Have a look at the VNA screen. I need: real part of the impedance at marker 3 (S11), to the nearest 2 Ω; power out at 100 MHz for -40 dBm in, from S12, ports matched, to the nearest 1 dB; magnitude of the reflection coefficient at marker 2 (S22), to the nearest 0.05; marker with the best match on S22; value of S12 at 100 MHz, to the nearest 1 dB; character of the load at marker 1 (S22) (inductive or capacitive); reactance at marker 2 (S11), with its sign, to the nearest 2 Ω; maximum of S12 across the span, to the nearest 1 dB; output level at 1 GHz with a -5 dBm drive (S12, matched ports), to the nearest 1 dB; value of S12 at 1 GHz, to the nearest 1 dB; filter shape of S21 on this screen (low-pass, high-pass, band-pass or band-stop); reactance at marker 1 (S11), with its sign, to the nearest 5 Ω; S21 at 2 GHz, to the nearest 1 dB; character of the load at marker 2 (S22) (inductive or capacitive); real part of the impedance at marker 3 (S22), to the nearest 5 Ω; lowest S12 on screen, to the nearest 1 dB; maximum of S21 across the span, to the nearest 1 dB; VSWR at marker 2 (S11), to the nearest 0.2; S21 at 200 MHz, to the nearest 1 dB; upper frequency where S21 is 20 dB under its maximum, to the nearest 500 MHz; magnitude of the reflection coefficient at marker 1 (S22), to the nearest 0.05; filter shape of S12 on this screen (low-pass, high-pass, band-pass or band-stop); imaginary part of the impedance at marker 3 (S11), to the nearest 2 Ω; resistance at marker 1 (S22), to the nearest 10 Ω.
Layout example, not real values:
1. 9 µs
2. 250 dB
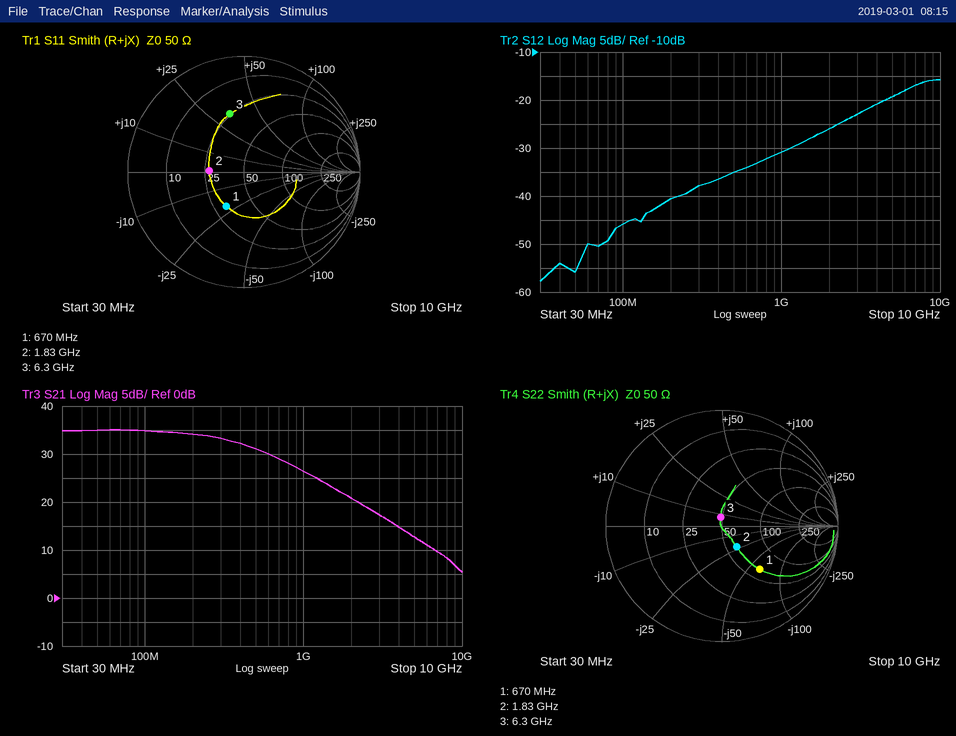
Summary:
1. 24 Ω
2. -86 dBm
3. 0.20
4. marker 3
5. -46 dB
6. capacitive
7. 0 Ω
8. -16 dB
9. -36 dBm
10. -31 dB
11. low-pass
12. -20 Ω
13. 21 dB
14. capacitive
15. 50 Ω
16. -58 dB
17. 35 dB
18. 1.8
19. 34 dB
20. 4.0 GHz
21. 0.50
22. high-pass
23. +34 Ω
24. 60 Ω
